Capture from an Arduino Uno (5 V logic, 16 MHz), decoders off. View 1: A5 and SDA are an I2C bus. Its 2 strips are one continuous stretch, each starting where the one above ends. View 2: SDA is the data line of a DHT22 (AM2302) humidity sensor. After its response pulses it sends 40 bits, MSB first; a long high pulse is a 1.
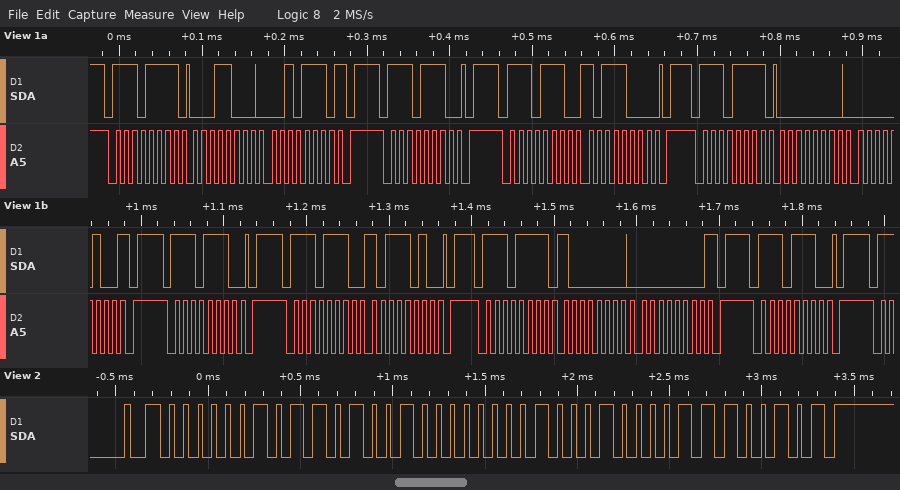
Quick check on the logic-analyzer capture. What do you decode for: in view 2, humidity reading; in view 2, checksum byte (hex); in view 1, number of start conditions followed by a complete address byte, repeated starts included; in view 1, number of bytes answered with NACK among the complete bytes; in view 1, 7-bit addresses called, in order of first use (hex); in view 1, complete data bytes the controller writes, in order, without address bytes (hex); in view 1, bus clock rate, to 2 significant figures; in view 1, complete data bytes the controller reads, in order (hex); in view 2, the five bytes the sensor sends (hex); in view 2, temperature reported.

72.2 %
0xE5
8
3
0x77
B8 BA
100 kHz
18 2E 00 04 80 00
02 D2 01 10 E5
27.2 °C
